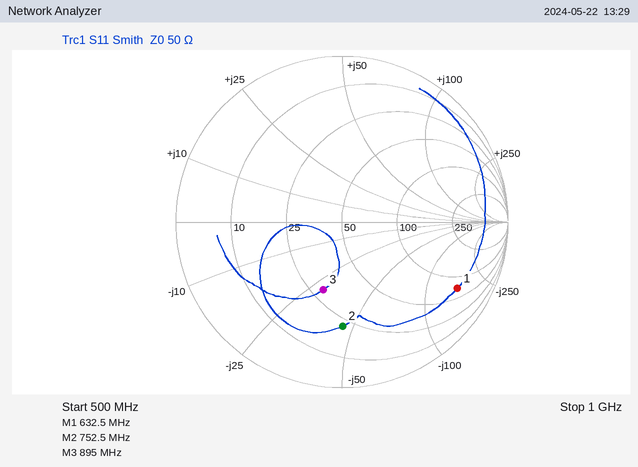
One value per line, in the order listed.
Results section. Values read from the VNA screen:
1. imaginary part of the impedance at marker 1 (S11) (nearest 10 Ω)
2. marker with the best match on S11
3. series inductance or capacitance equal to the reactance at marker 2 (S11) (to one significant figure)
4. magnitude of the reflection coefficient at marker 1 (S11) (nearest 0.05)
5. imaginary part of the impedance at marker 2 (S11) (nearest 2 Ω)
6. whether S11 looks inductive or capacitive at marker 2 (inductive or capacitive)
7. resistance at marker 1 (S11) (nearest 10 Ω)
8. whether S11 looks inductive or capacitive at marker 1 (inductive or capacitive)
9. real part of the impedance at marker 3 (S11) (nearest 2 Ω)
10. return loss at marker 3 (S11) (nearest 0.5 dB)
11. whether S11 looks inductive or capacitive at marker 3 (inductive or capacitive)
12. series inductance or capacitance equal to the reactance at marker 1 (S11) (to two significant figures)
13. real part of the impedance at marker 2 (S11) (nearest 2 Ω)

-160 Ω
marker 3
5 pF
0.80
-46 Ω
capacitive
70 Ω
capacitive
30 Ω
7.5 dB
capacitive
1.6 pF
22 Ω
